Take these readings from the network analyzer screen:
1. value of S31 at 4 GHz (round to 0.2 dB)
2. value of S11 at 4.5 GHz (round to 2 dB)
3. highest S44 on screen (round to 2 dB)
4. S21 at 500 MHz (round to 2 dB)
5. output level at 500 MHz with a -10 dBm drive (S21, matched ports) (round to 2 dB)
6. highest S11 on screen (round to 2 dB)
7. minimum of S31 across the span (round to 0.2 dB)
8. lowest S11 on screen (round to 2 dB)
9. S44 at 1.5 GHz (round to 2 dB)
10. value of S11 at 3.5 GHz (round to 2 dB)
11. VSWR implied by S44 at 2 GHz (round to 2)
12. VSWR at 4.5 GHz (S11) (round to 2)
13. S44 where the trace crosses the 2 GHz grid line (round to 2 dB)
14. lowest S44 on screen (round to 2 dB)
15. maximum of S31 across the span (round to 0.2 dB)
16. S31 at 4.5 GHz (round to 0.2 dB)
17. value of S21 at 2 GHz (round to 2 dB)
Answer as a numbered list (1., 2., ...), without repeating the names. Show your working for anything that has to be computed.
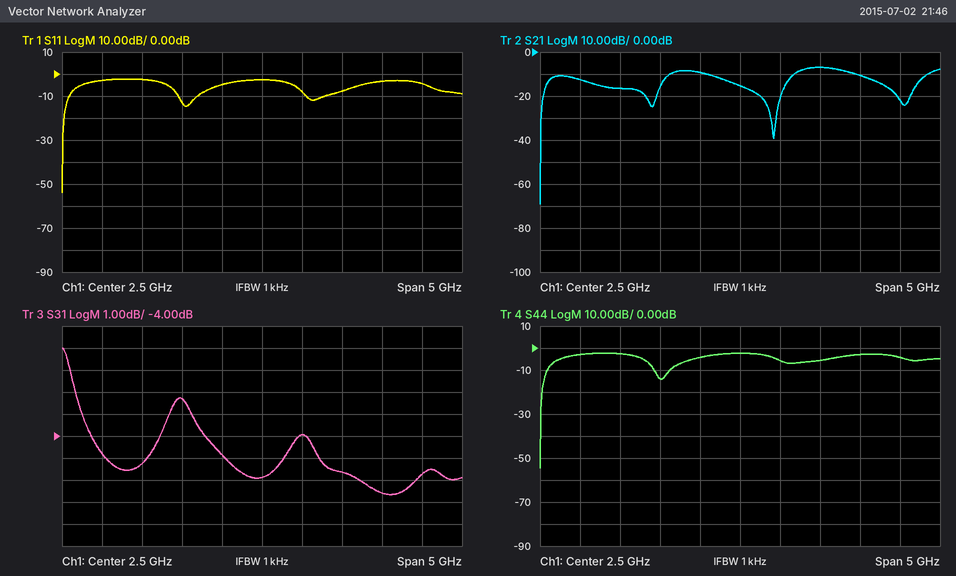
1. -6.6 dB
2. -4 dB
3. -2 dB
4. -12 dB
5. -10 dBm + (-12 dB) = -22 dBm
6. -2 dB
7. -6.6 dB
8. -54 dB
9. -14 dB
10. -8 dB
11. |Γ| = 10^(-4/20) = 0.6310; VSWR = (1 + 0.6310)/(1 − 0.6310) ≈ 4
12. |Γ| = 10^(-4/20) = 0.6310; VSWR = (1 + 0.6310)/(1 − 0.6310) ≈ 4
13. -4 dB
14. -54 dB
15. 0.0 dB
16. -5.8 dB
17. -10 dB
